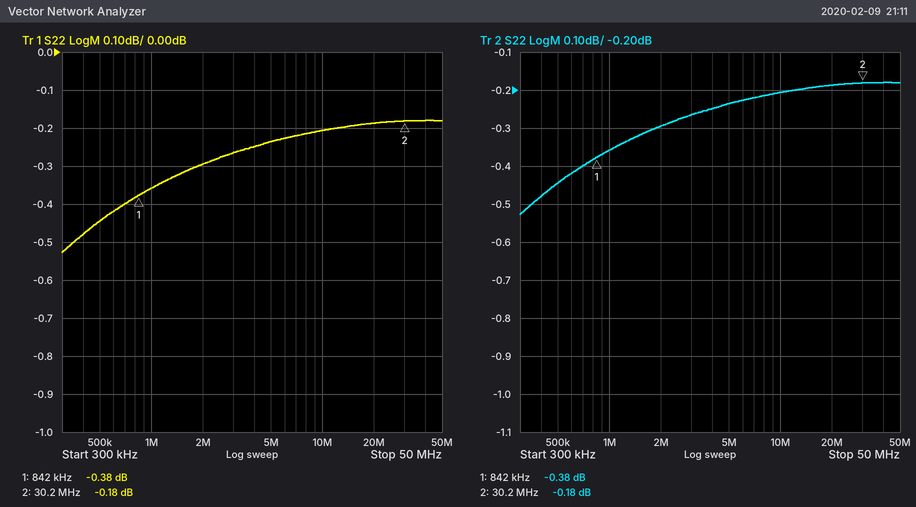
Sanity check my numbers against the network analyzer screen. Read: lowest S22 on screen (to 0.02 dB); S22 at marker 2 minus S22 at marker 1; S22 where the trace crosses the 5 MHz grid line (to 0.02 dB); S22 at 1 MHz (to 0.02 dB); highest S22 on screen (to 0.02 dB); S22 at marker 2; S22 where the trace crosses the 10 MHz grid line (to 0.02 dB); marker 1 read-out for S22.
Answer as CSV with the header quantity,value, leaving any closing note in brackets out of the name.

quantity,value
lowest S22 on screen,-0.52 dB
S22 at marker 2 minus S22 at marker 1,0.20 dB
S22 where the trace crosses the 5 MHz grid line,-0.24 dB
S22 at 1 MHz,-0.36 dB
highest S22 on screen,-0.18 dB
S22 at marker 2,-0.18 dB
S22 where the trace crosses the 10 MHz grid line,-0.20 dB
marker 1 read-out for S22,-0.38 dB
